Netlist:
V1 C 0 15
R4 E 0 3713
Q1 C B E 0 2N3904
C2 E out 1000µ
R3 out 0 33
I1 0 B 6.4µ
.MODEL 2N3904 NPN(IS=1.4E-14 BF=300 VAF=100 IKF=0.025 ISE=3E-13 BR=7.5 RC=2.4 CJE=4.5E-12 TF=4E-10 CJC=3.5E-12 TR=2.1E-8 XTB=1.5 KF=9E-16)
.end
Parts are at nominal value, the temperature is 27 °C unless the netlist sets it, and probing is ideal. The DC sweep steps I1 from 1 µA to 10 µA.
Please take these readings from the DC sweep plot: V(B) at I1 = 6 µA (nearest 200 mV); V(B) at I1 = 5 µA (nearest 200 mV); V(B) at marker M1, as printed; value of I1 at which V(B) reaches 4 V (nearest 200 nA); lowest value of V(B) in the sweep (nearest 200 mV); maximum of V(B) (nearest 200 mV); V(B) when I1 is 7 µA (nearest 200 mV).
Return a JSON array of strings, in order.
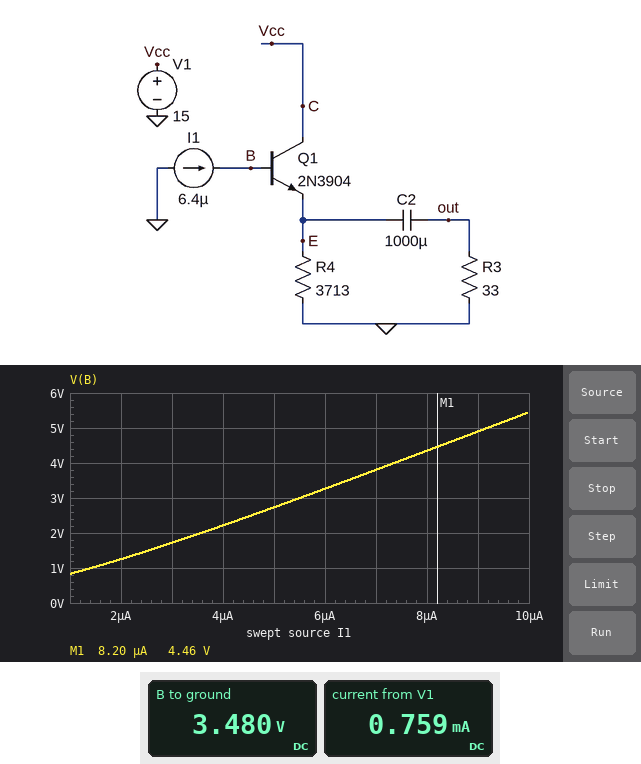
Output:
["3.2 V", "2.8 V", "4.46 V", "7.4 µA", "800 mV", "5.4 V", "3.8 V"]
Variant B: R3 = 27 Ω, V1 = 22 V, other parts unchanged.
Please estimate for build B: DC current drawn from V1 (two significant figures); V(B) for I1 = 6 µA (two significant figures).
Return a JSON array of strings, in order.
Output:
["810 µA", "3.4 V"]
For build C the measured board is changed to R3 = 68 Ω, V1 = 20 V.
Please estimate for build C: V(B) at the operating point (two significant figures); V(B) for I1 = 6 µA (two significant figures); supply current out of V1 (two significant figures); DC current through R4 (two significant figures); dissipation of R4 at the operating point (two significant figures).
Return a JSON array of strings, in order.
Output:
["3.6 V", "3.4 V", "790 µA", "800 µA", "2.4 mW"]
